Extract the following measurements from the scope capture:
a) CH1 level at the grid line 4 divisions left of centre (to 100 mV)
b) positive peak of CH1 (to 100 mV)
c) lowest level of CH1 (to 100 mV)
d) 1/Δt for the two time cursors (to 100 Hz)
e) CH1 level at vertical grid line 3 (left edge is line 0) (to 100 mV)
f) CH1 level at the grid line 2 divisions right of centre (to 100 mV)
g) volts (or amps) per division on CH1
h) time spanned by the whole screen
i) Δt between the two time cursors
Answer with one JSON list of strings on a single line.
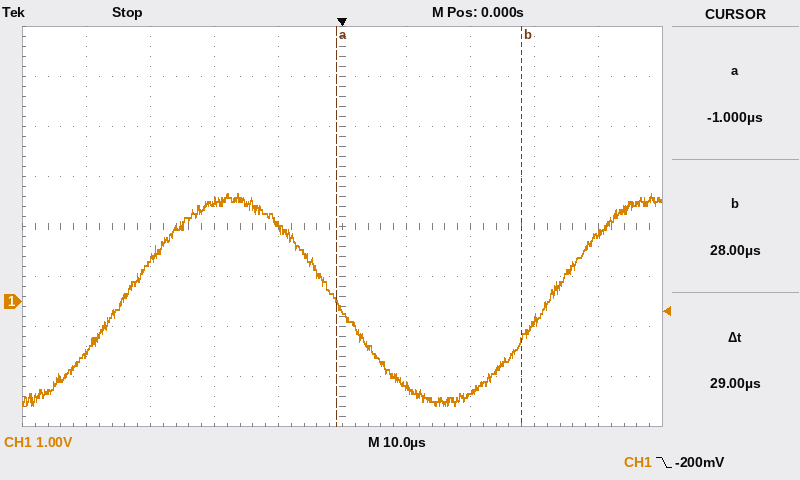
["-1.0 V", "2.2 V", "-2.1 V", "34.5 kHz", "2.0 V", "-1.8 V", "1 V", "100 µs", "29 µs"]
